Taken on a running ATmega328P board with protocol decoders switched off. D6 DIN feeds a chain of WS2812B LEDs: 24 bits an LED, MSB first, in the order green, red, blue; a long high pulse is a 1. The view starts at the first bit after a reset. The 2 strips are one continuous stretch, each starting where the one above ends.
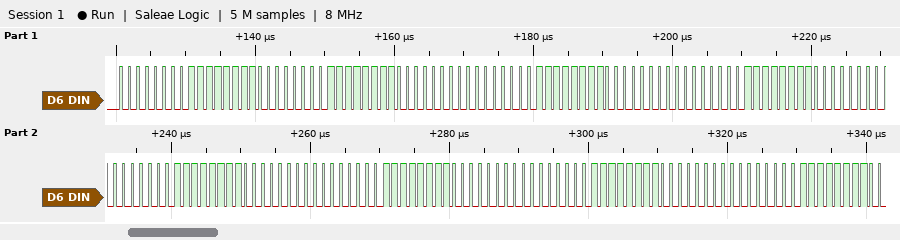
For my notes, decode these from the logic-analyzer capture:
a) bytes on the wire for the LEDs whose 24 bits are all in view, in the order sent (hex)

00 FF 00 FF 00 00 FF 00 00 FF 00 00 FF 00 00 FF 00 00 FF 00 00
